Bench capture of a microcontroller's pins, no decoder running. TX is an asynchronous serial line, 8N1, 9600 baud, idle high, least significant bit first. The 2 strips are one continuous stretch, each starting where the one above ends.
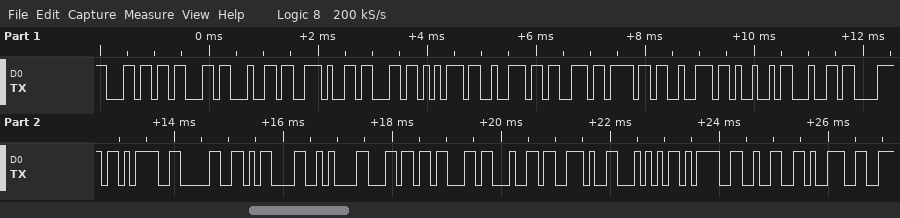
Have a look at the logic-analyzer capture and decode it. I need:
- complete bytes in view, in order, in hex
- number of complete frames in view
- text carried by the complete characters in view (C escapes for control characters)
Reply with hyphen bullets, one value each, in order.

- 6C 63 64 2E 63 75 72 73 6F 72 49 64 78 3D 30 0D 0A 6C 63 64 2E 54 3D 32 39
- 25
- "lcd.cursorIdx=0\r\nlcd.T=29"
